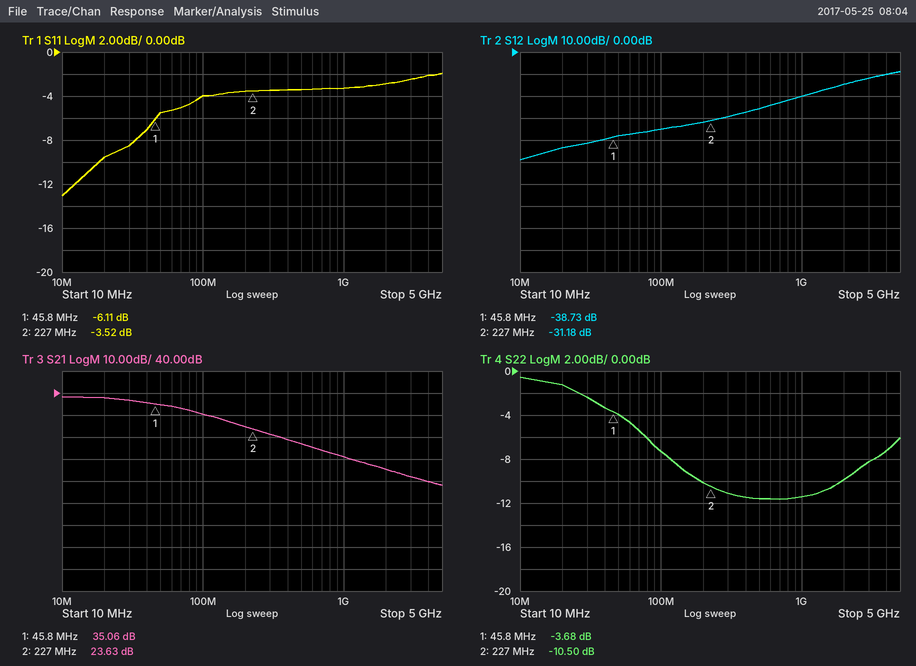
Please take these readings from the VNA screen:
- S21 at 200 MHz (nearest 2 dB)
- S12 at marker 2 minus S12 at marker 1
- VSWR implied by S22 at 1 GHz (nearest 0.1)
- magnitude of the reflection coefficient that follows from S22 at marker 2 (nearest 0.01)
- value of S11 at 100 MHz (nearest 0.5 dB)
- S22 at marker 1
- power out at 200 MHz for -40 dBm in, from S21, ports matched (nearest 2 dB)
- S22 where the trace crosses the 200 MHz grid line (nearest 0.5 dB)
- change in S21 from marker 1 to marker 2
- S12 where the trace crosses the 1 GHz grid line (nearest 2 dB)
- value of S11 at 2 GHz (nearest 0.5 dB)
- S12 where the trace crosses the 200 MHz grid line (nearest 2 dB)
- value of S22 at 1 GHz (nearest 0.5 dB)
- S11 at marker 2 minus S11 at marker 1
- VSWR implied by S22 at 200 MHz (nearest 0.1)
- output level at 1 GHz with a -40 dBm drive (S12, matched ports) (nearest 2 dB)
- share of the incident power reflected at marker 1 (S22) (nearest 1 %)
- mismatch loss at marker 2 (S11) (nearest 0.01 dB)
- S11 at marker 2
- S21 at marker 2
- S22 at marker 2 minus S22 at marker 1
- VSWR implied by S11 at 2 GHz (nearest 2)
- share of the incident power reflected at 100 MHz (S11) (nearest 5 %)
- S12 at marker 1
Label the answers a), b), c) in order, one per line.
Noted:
a) 24 dB
b) 7.55 dB
c) 1.7
d) 0.30
e) -4.0 dB
f) -3.68 dB
g) -16 dBm
h) -10.0 dB
i) -11.43 dB
j) -20 dB
k) -3.0 dB
l) -32 dB
m) -11.5 dB
n) 2.59 dB
o) 1.9
p) -60 dBm
q) 43 %
r) 2.55 dB
s) -3.52 dB
t) 23.63 dB
u) -6.82 dB
v) 6
w) 40 %
x) -38.73 dB
